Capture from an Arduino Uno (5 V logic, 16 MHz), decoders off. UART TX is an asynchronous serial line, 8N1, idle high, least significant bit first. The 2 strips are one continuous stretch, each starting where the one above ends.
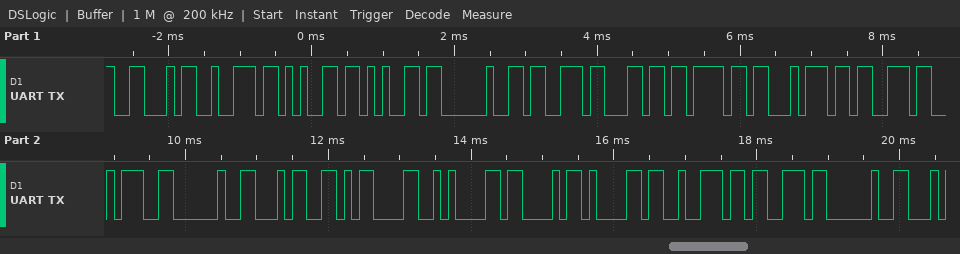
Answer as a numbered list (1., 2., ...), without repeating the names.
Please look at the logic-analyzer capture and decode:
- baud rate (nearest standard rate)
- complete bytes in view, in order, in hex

1. 9600 baud
2. 0x46 0x72 0x65 0x65 0x20 0x73 0x6C 0x6F 0x74 0x73 0x3A 0x20 0x34 0x0D 0x0A 0x43 0x61 0x72 0x73 0x20
